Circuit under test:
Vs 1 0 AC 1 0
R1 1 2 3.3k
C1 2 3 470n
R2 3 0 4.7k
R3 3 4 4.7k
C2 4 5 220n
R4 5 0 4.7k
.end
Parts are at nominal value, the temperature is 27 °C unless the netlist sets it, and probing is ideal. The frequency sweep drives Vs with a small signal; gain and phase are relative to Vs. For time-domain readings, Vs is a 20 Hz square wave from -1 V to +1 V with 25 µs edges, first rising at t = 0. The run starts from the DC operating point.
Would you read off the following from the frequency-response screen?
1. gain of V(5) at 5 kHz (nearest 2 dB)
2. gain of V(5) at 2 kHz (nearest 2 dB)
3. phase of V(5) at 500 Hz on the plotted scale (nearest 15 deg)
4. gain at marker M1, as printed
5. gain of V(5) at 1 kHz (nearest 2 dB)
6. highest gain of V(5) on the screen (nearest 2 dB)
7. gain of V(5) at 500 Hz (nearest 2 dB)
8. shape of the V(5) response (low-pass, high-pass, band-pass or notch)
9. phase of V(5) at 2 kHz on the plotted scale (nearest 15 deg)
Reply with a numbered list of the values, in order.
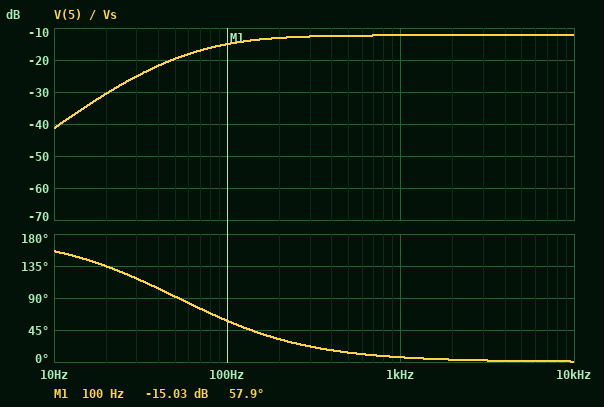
1. -12 dB
2. -12 dB
3. 15 deg
4. -15.03 dB
5. -12 dB
6. -12 dB
7. -12 dB
8. high-pass
9. 0 deg
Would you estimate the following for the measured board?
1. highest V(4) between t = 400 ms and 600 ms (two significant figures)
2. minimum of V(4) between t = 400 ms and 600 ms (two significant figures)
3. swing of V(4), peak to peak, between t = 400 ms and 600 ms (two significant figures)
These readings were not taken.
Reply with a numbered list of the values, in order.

1. 540 mV
2. -540 mV
3. 1.1 V
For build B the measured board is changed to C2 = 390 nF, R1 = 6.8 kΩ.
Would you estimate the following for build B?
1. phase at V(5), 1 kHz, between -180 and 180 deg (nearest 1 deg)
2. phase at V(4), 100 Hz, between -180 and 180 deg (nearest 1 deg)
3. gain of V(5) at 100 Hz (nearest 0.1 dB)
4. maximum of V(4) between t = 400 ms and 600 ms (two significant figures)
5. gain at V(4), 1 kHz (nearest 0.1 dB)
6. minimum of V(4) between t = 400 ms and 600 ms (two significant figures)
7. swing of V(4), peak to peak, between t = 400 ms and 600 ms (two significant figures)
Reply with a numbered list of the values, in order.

1. 4 deg
2. -4 deg
3. -17.1 dB
4. 330 mV
5. -16.0 dB
6. -330 mV
7. 650 mV
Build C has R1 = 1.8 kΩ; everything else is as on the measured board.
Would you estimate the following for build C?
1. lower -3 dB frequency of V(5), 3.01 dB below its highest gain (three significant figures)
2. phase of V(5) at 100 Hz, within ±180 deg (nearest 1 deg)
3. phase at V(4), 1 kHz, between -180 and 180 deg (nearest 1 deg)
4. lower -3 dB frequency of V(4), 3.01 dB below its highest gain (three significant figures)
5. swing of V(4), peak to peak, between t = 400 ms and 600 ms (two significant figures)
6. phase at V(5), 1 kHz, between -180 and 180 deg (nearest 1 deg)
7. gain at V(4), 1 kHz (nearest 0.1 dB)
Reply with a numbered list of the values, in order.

1. 112 Hz
2. 65 deg
3. -1 deg
4. 24.9 Hz
5. 1.3 V
6. 8 deg
7. -9.9 dB
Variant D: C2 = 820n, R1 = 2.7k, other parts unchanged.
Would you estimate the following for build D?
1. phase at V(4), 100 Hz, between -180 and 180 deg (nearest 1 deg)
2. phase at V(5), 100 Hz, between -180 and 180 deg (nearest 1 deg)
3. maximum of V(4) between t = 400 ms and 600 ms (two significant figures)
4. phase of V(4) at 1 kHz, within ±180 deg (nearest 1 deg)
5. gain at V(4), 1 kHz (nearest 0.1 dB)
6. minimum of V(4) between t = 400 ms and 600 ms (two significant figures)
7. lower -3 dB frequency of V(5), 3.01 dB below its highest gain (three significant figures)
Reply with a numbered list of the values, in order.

1. 17 deg
2. 39 deg
3. 500 mV
4. 2 deg
5. -11.4 dB
6. -500 mV
7. 65.2 Hz
